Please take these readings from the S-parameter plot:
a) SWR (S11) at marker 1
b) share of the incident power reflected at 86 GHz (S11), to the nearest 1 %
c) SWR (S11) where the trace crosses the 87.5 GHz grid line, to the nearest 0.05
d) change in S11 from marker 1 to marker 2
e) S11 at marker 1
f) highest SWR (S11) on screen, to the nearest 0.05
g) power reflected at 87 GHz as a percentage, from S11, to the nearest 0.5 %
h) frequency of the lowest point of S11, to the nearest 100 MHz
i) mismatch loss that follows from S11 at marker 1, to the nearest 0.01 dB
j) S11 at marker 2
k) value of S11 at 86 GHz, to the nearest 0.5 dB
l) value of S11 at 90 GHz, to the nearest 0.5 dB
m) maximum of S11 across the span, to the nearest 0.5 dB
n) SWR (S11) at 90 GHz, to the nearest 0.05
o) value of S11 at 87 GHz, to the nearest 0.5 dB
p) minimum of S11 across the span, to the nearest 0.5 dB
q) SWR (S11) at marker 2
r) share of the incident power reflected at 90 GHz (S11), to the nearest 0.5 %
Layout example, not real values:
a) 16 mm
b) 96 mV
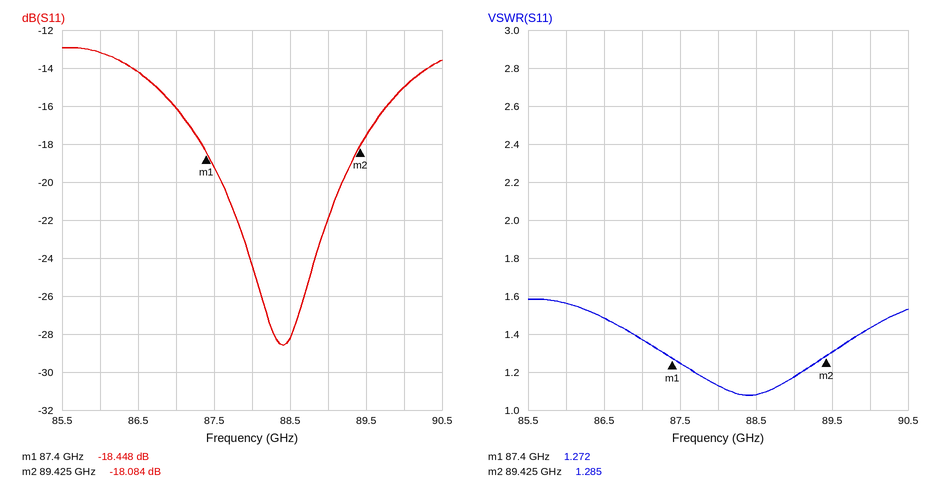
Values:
a) 1.272
b) 5 %
c) 1.25
d) 0.364 dB
e) -18.448 dB
f) 1.60
g) 2.5 %
h) 88.4 GHz
i) 0.06 dB
j) -18.084 dB
k) -13.0 dB
l) -15.0 dB
m) -13.0 dB
n) 1.45
o) -16.0 dB
p) -28.5 dB
q) 1.285
r) 3.0 %
